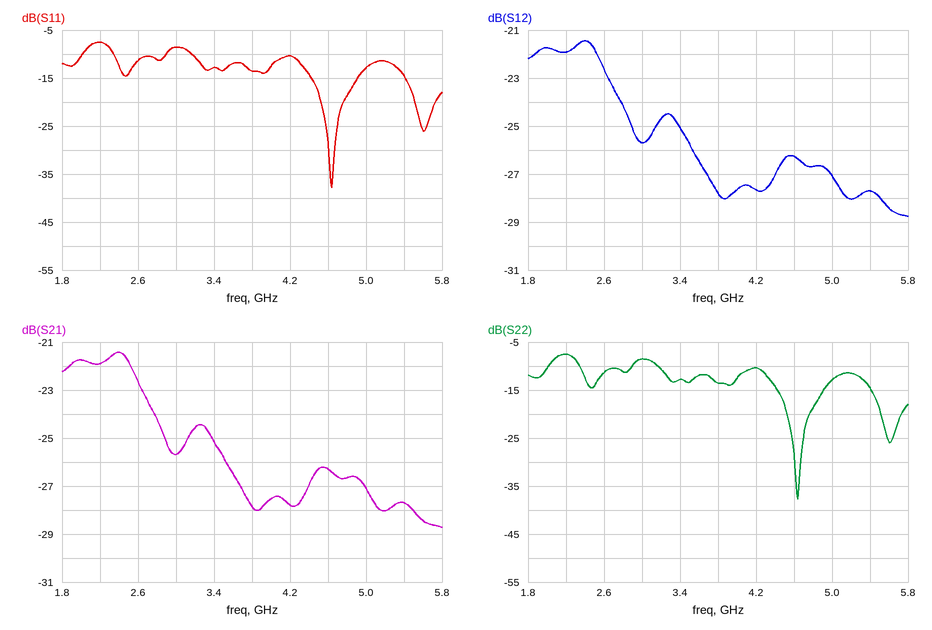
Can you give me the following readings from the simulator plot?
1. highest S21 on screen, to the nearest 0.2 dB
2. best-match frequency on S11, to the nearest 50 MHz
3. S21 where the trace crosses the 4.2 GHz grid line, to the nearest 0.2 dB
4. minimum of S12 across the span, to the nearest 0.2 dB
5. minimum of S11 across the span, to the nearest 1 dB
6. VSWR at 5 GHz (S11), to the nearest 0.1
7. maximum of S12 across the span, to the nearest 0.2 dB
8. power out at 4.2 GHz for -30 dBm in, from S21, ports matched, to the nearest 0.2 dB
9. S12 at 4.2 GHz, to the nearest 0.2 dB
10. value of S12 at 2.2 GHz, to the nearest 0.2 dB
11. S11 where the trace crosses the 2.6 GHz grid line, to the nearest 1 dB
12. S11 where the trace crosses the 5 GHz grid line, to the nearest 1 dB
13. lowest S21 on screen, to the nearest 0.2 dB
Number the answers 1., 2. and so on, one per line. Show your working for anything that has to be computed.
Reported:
1. -21.4 dB
2. 4.65 GHz
3. -27.8 dB
4. -28.8 dB
5. -38 dB
6. |Γ| = 10^(-13/20) = 0.2239; VSWR = (1 + 0.2239)/(1 − 0.2239) ≈ 1.6
7. -21.4 dB
8. -30 dBm + (-27.8 dB) = -57.8 dBm
9. -27.6 dB
10. -22.0 dB
11. -11 dB
12. -13 dB
13. -28.8 dB
